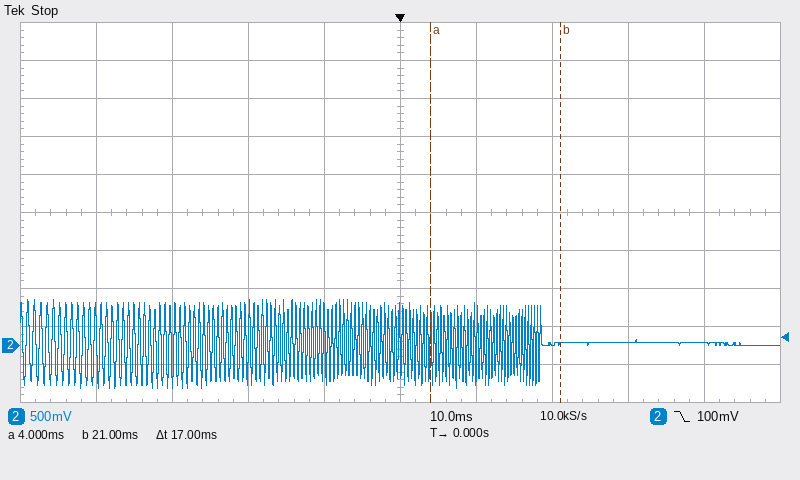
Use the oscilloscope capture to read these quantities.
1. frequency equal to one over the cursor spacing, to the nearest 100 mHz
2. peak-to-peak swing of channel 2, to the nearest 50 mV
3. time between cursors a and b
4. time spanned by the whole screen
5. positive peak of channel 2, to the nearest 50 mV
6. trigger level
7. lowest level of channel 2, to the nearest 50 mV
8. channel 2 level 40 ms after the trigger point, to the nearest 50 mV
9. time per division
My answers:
58.8 Hz
1.15 V
17 ms
100 ms
600 mV
100 mV
-550 mV
50 mV
10 ms
